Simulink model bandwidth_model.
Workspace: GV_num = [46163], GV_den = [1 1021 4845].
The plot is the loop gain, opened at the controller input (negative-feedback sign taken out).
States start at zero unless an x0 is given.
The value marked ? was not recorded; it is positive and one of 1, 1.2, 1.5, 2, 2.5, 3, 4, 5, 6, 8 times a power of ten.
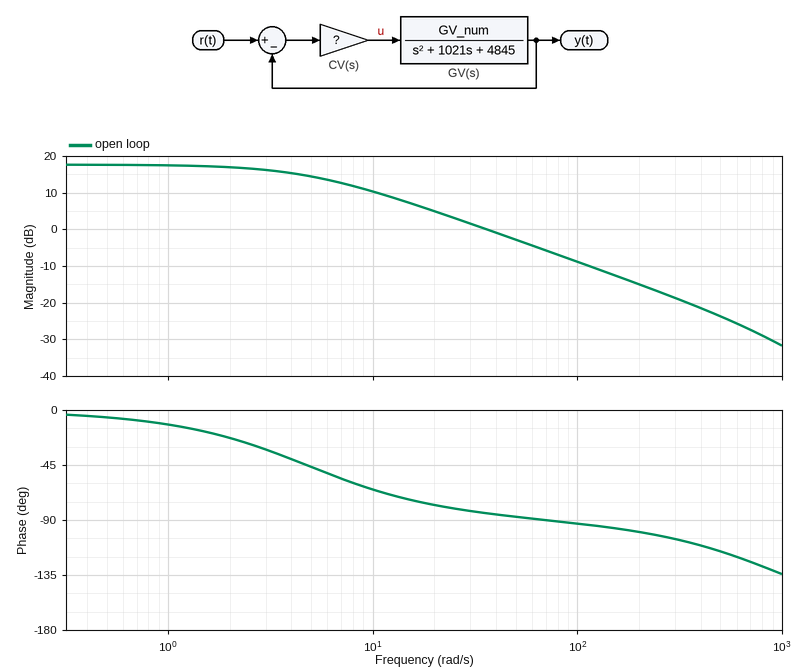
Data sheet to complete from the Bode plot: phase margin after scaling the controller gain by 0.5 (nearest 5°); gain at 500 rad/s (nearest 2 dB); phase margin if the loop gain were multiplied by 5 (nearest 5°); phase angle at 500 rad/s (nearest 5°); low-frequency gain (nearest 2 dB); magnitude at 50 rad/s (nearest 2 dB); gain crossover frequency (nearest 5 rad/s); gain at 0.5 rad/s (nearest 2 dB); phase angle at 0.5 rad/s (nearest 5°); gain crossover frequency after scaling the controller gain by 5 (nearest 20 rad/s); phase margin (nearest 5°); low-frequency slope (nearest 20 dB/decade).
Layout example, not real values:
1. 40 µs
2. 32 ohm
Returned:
1. 105°
2. -24 dB
3. 80°
4. -115°
5. 18 dB
6. -2 dB
7. 35 rad/s
8. 18 dB
9. -5°
10. 180 rad/s
11. 95°
12. 0 dB/decade
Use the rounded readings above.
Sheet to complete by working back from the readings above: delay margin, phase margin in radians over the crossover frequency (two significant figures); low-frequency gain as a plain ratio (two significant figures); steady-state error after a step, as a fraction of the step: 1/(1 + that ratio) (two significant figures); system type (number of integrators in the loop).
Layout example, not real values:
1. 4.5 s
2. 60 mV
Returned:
1. 0.047 s
2. 7.9
3. 0.11
4. 0
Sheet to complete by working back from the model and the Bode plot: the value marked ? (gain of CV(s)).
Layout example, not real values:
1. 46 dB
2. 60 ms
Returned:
1. 0.8
